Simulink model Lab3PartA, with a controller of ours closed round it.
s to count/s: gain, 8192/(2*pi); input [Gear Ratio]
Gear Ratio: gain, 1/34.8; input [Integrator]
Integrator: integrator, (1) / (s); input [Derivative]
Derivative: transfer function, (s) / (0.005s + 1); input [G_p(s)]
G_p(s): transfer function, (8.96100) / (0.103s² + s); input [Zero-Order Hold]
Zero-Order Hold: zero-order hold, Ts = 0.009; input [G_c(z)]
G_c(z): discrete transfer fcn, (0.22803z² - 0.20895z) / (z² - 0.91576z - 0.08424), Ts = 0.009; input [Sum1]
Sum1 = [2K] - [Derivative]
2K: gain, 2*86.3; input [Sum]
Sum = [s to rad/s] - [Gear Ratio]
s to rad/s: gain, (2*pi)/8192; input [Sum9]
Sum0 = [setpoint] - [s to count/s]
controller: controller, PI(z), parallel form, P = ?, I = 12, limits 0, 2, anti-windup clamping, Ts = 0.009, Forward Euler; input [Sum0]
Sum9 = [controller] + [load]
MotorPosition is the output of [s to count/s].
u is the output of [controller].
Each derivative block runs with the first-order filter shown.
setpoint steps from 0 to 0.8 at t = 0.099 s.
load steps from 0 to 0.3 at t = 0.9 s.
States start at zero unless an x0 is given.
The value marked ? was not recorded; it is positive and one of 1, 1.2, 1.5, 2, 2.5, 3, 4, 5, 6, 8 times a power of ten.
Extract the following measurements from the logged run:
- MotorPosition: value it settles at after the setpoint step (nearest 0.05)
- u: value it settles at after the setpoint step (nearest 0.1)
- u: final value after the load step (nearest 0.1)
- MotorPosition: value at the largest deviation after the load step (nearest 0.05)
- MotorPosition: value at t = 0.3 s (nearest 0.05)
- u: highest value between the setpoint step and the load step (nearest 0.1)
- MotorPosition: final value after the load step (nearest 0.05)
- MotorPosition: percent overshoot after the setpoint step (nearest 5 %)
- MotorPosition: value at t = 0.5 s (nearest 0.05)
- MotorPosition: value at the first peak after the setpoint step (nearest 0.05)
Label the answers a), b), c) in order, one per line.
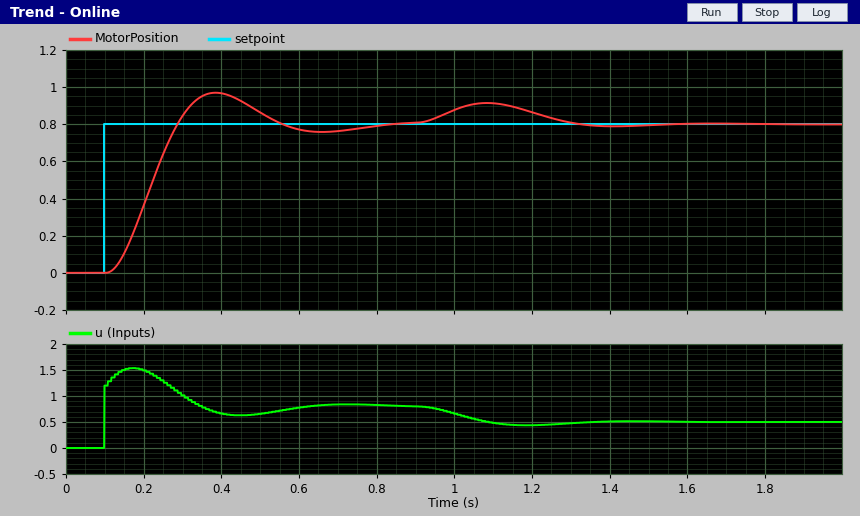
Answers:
a) 0.80
b) 0.8
c) 0.5
d) 0.90
e) 0.85
f) 1.5
g) 0.80
h) 20 %
i) 0.85
j) 0.95
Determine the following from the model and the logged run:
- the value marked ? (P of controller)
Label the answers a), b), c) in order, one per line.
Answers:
a) 1.5
